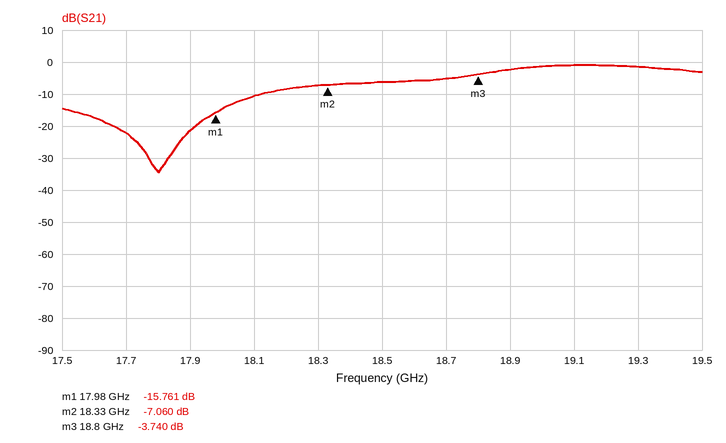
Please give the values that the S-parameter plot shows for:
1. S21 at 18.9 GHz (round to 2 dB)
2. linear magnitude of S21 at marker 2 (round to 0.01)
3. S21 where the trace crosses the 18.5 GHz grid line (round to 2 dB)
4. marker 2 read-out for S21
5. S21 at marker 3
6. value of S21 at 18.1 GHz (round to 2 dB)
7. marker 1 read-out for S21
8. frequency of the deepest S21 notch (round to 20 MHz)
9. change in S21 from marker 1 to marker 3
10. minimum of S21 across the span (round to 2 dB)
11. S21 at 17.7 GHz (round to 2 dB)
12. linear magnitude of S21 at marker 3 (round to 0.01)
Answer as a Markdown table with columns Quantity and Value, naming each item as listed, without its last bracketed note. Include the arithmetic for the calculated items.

| Quantity | Value |
|---|---|
| S21 at 18.9 GHz | -2 dB |
| linear magnitude of S21 at marker 2 | 10^(-7.06/20) ≈ 0.44 |
| S21 where the trace crosses the 18.5 GHz grid line | -6 dB |
| marker 2 read-out for S21 | -7.060 dB |
| S21 at marker 3 | -3.740 dB |
| value of S21 at 18.1 GHz | -10 dB |
| marker 1 read-out for S21 | -15.761 dB |
| frequency of the deepest S21 notch | 17.80 GHz |
| change in S21 from marker 1 to marker 3 | -3.74 − (-15.761) = 12.021 dB |
| minimum of S21 across the span | -34 dB |
| S21 at 17.7 GHz | -22 dB |
| linear magnitude of S21 at marker 3 | 10^(-3.74/20) ≈ 0.65 |
